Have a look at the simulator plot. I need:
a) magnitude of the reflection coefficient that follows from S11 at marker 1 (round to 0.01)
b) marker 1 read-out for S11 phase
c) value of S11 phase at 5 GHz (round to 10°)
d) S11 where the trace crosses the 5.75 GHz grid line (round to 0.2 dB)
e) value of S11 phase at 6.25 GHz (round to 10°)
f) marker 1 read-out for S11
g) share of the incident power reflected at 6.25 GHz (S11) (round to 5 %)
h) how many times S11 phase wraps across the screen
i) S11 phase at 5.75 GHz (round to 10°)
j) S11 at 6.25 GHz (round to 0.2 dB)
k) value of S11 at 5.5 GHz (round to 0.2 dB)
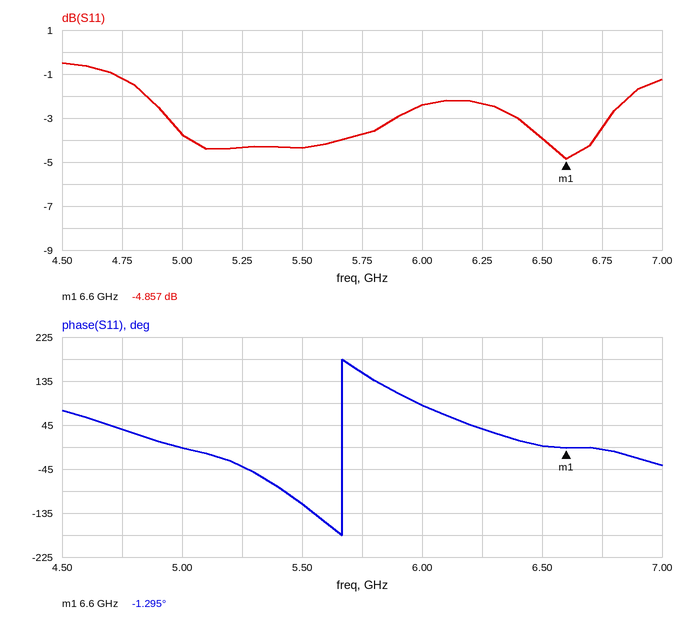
0.57
-1.295°
0°
-3.8 dB
40°
-4.857 dB
60 %
1
150°
-2.4 dB
-4.4 dB
